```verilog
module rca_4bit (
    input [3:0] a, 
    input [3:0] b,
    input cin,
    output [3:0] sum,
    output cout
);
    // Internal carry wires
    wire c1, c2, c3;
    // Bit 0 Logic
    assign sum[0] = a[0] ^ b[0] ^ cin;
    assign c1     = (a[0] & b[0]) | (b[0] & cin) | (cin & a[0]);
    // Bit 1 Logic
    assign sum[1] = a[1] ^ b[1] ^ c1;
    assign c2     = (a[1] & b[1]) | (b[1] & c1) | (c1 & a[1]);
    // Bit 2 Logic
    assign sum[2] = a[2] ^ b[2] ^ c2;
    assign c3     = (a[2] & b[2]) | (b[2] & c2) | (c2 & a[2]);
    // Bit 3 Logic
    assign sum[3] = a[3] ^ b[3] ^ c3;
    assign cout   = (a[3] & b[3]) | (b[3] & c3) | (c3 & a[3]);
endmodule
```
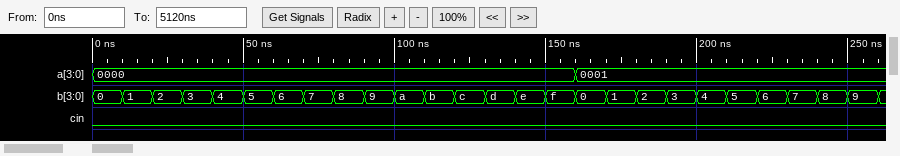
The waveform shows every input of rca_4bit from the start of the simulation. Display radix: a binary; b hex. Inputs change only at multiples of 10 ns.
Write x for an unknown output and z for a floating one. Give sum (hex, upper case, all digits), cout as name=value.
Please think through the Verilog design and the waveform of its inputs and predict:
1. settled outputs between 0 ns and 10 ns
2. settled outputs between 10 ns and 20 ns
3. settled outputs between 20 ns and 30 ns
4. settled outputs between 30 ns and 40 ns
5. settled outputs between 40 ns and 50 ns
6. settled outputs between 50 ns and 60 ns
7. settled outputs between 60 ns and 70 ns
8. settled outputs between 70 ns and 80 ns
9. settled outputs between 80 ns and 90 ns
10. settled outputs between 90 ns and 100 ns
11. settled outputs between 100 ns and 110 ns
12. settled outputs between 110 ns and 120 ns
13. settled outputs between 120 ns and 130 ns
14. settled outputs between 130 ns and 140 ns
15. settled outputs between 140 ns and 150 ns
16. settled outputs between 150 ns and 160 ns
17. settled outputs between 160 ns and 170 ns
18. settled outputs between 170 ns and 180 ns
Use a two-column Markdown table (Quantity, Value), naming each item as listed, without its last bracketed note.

| Quantity | Value |
|---|---|
| settled outputs between 0 ns and 10 ns | sum=0, cout=0 |
| settled outputs between 10 ns and 20 ns | sum=1, cout=0 |
| settled outputs between 20 ns and 30 ns | sum=2, cout=0 |
| settled outputs between 30 ns and 40 ns | sum=3, cout=0 |
| settled outputs between 40 ns and 50 ns | sum=4, cout=0 |
| settled outputs between 50 ns and 60 ns | sum=5, cout=0 |
| settled outputs between 60 ns and 70 ns | sum=6, cout=0 |
| settled outputs between 70 ns and 80 ns | sum=7, cout=0 |
| settled outputs between 80 ns and 90 ns | sum=8, cout=0 |
| settled outputs between 90 ns and 100 ns | sum=9, cout=0 |
| settled outputs between 100 ns and 110 ns | sum=A, cout=0 |
| settled outputs between 110 ns and 120 ns | sum=B, cout=0 |
| settled outputs between 120 ns and 130 ns | sum=C, cout=0 |
| settled outputs between 130 ns and 140 ns | sum=D, cout=0 |
| settled outputs between 140 ns and 150 ns | sum=E, cout=0 |
| settled outputs between 150 ns and 160 ns | sum=F, cout=0 |
| settled outputs between 160 ns and 170 ns | sum=1, cout=0 |
| settled outputs between 170 ns and 180 ns | sum=2, cout=0 |
